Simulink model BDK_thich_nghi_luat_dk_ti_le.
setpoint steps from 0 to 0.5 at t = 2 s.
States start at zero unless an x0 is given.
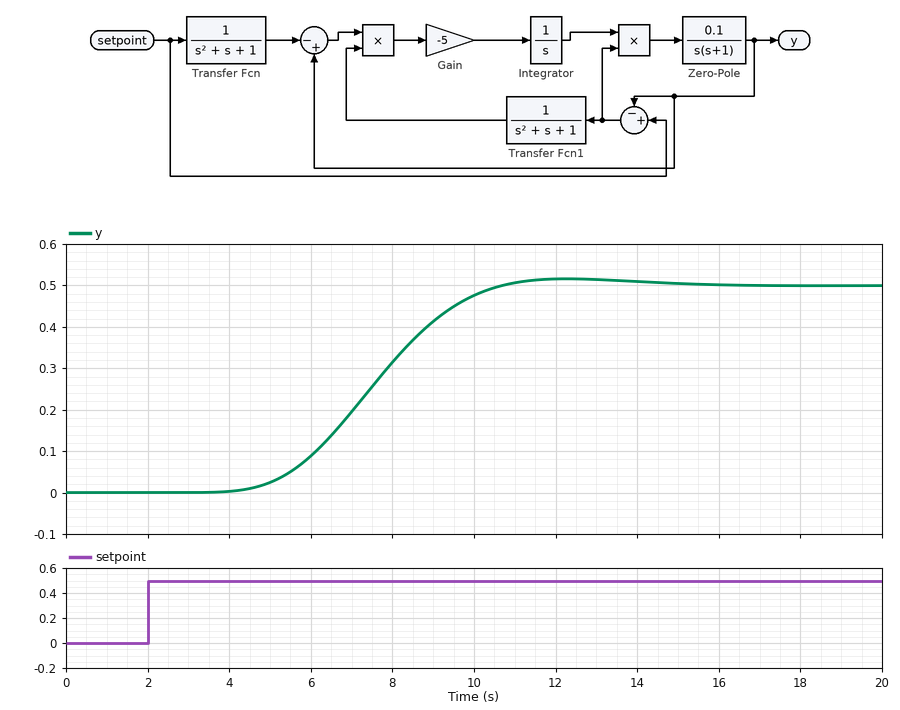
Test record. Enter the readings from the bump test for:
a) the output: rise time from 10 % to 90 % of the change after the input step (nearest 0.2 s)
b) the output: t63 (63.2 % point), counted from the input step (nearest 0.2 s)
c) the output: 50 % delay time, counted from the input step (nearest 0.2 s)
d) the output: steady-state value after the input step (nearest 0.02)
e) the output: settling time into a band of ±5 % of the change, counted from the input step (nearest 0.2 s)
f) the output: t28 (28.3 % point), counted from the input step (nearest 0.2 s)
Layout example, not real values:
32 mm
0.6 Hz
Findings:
4.0 s
6.0 s
5.4 s
0.50
8.0 s
4.6 s
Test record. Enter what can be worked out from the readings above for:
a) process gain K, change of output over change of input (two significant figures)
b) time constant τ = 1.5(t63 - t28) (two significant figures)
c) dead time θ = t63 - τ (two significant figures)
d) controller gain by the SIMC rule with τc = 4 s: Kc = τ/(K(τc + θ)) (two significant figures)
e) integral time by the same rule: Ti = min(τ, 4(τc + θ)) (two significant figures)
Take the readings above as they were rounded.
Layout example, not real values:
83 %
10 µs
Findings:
1.0
2.1 s
3.9 s
0.27
2.1 s
